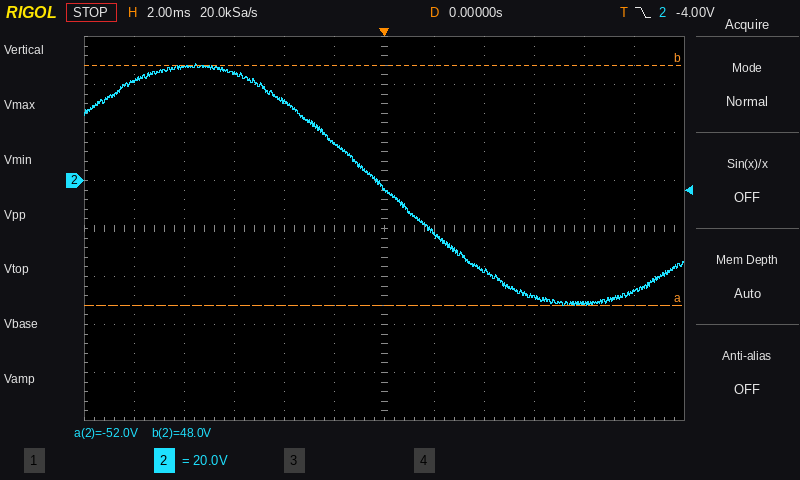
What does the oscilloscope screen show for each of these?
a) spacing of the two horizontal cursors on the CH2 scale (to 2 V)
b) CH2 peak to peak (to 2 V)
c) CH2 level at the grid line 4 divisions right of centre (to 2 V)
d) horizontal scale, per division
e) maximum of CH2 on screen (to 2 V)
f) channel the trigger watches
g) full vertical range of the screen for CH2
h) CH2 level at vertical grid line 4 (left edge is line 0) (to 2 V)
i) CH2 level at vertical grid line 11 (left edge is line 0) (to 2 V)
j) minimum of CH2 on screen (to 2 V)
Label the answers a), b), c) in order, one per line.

a) 100 V
b) 100 V
c) -52 V
d) 2 ms
e) 48 V
f) CH2
g) 160 V
h) 34 V
i) -46 V
j) -52 V
